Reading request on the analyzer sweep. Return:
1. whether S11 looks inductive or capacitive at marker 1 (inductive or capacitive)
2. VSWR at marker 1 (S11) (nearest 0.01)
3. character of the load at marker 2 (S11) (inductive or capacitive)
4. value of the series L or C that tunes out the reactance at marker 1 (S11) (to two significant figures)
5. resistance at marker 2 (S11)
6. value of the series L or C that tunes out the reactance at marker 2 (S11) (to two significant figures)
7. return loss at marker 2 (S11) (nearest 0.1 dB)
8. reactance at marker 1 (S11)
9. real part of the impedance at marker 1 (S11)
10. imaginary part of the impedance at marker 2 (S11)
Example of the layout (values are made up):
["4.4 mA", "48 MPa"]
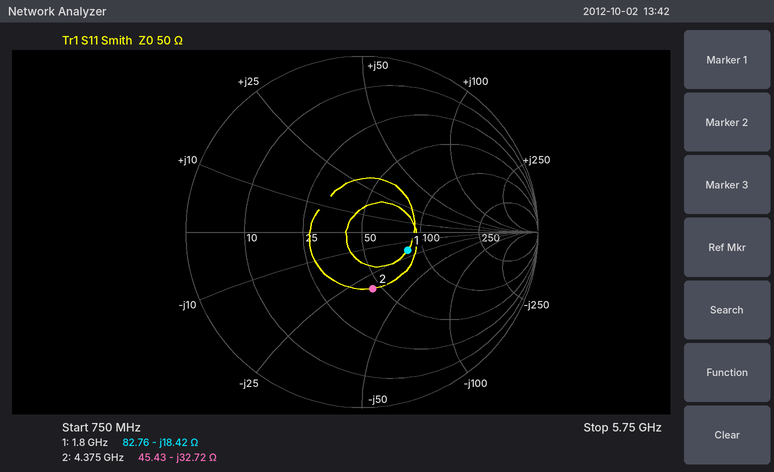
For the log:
["capacitive", "1.78", "capacitive", "1.6 nH", "45.43 Ω", "1.2 nH", "9.7 dB", "-18.42 Ω", "82.76 Ω", "-32.72 Ω"]
